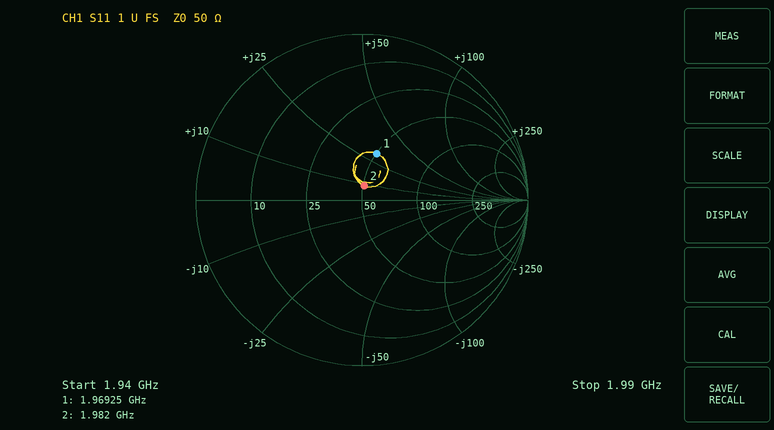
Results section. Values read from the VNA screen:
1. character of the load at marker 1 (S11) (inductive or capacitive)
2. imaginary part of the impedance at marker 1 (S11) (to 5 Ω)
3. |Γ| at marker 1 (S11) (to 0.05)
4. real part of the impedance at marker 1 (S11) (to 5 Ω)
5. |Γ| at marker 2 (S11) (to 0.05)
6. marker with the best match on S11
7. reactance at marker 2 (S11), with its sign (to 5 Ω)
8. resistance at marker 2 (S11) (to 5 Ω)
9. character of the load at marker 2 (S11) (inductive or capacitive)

inductive
+30 Ω
0.30
50 Ω
0.10
marker 2
+10 Ω
50 Ω
inductive
